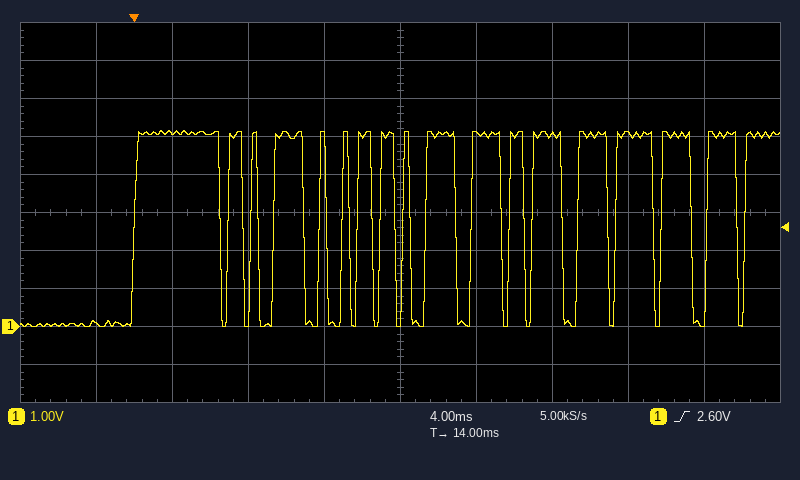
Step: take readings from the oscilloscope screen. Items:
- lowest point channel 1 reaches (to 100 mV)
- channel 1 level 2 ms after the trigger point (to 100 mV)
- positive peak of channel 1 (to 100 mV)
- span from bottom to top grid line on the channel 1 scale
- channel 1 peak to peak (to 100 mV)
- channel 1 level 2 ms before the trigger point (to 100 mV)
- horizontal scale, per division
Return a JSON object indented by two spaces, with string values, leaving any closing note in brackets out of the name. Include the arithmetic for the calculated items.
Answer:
{
  "lowest point channel 1 reaches": "0.0 V",
  "channel 1 level 2 ms after the trigger point": "5.1 V",
  "positive peak of channel 1": "5.2 V",
  "span from bottom to top grid line on the channel 1 scale": "10 V",
  "channel 1 peak to peak": "5.2 V − (0.0 V) = 5.2 V",
  "channel 1 level 2 ms before the trigger point": "100 mV",
  "horizontal scale, per division": "4 ms"
}
